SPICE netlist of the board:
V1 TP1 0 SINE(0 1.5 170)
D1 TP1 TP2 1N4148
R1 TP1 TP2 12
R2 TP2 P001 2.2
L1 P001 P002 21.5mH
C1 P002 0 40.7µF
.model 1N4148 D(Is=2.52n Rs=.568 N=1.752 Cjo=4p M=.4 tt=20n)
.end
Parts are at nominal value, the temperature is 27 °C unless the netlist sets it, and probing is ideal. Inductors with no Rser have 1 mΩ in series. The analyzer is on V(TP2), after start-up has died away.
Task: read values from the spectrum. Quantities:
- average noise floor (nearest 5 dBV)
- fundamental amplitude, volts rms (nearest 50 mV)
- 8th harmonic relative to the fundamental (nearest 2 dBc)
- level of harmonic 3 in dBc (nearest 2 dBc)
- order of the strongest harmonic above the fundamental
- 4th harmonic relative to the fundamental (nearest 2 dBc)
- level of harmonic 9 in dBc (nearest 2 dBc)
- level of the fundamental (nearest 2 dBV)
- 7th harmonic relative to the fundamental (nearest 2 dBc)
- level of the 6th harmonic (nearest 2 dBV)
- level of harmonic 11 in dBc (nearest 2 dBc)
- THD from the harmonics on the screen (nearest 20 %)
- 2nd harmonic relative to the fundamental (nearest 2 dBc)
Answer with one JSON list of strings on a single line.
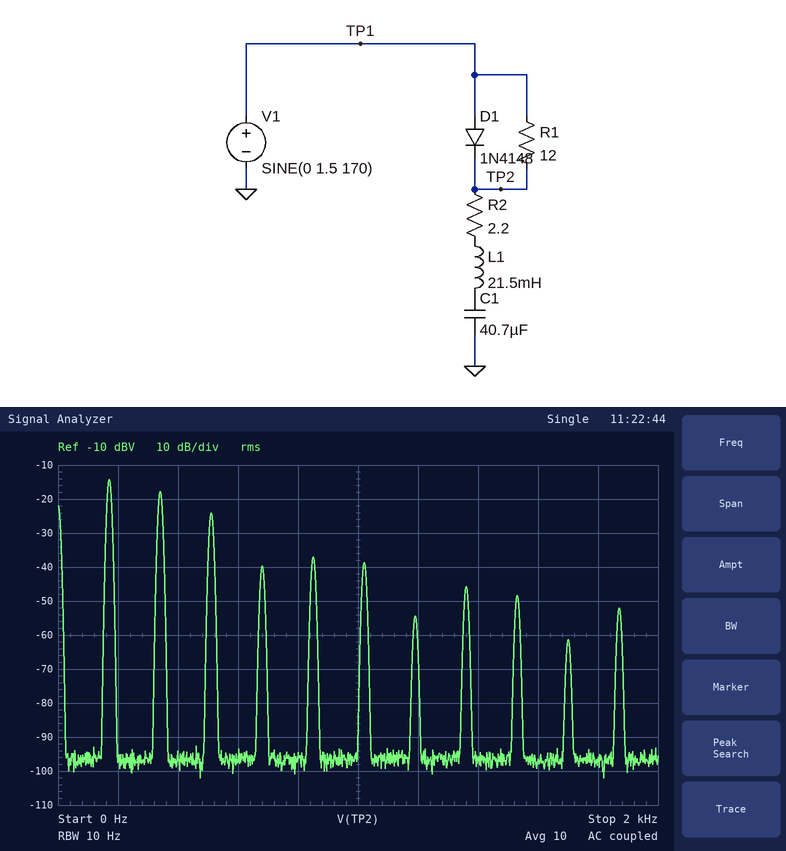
["-95 dBV", "200 mV", "-32 dBc", "-10 dBc", "2", "-26 dBc", "-34 dBc", "-14 dBV", "-40 dBc", "-38 dBV", "-38 dBc", "80 %", "-4 dBc"]
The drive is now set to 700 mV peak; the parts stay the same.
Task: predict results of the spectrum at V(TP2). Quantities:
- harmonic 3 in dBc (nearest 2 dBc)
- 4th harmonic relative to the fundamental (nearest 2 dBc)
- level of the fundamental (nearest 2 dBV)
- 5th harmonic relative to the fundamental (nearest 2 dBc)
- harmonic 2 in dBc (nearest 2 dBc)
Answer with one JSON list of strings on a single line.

["-36 dBc", "-38 dBc", "-22 dBV", "-42 dBc", "-34 dBc"]
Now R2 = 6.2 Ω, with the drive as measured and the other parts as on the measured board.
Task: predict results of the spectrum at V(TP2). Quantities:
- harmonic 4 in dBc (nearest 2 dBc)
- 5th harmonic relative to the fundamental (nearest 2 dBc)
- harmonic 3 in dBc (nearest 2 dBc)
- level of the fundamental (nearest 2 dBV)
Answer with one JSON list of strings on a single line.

["-28 dBc", "-46 dBc", "-20 dBc", "-8 dBV"]
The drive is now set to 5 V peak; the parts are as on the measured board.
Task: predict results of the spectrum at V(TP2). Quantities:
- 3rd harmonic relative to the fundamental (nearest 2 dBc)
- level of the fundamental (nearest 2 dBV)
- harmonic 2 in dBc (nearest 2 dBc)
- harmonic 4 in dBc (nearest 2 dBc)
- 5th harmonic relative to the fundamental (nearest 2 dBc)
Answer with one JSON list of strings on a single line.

["-16 dBc", "-2 dBV", "0 dBc", "-14 dBc", "-22 dBc"]
